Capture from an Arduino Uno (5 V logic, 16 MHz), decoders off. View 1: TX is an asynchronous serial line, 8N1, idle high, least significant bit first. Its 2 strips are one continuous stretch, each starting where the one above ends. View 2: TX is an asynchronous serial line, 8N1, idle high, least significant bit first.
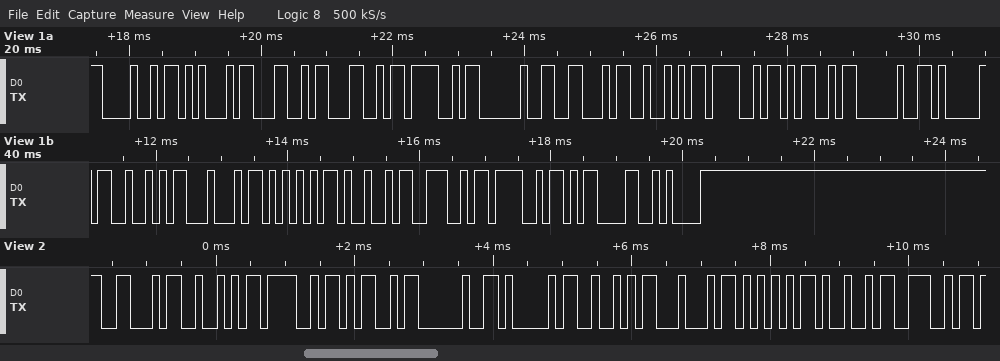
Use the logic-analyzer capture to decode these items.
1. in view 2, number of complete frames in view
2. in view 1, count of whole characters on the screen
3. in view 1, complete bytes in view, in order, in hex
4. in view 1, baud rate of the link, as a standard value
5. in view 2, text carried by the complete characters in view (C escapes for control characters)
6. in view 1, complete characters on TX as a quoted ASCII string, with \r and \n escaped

11
20
48 45 4C 4C 4F 20 46 52 4F 4D 20 41 52 44 55 49 4E 4F 0D 0A
9600 baud
"FROM ARDUIN"
"HELLO FROM ARDUINO\r\n"
